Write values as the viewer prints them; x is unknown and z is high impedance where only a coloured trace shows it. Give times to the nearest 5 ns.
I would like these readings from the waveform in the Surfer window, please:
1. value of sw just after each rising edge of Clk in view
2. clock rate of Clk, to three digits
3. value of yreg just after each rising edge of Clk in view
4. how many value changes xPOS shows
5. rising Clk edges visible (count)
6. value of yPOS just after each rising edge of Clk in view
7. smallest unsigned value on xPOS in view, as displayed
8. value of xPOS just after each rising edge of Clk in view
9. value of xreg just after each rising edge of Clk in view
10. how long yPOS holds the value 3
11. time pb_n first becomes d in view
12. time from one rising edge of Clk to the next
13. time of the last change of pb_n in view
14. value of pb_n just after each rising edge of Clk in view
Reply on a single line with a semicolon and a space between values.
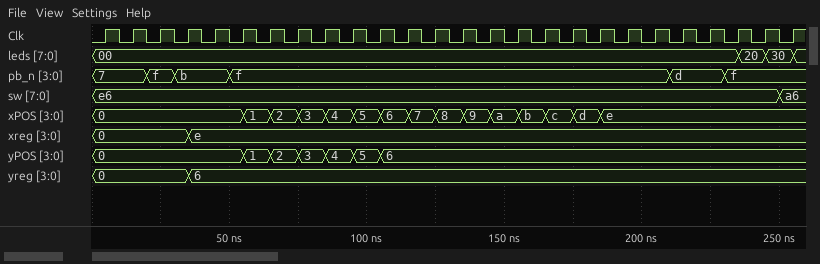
e6, e6, e6, e6, e6, e6, e6, e6, e6, e6, e6, e6, e6, e6, e6, e6, e6, e6, e6, e6, e6, e6, e6, e6, e6, a6; 100 MHz; 0, 0, 0, 6, 6, 6, 6, 6, 6, 6, 6, 6, 6, 6, 6, 6, 6, 6, 6, 6, 6, 6, 6, 6, 6, 6; 14; 26; 0, 0, 0, 0, 0, 1, 2, 3, 4, 5, 6, 6, 6, 6, 6, 6, 6, 6, 6, 6, 6, 6, 6, 6, 6, 6; 0; 0, 0, 0, 0, 0, 1, 2, 3, 4, 5, 6, 7, 8, 9, a, b, c, d, e, e, e, e, e, e, e, e; 0, 0, 0, e, e, e, e, e, e, e, e, e, e, e, e, e, e, e, e, e, e, e, e, e, e, e; 10 ns; 210 ns; 10 ns; 230 ns; 7, 7, f, b, b, f, f, f, f, f, f, f, f, f, f, f, f, f, f, f, f, d, d, f, f, f
